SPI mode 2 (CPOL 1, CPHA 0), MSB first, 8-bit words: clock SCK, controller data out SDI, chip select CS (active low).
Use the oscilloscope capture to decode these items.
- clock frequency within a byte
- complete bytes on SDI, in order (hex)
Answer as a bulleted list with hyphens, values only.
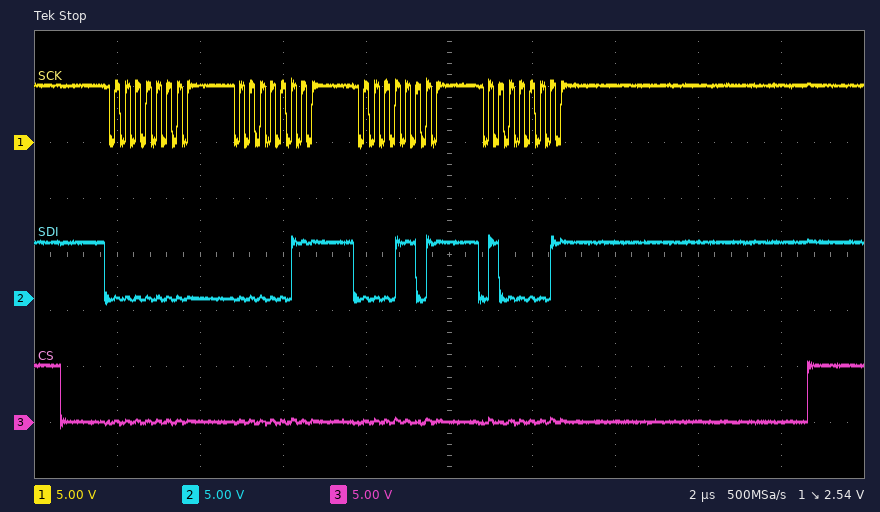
- 4 MHz
- 00 03 0D 41
